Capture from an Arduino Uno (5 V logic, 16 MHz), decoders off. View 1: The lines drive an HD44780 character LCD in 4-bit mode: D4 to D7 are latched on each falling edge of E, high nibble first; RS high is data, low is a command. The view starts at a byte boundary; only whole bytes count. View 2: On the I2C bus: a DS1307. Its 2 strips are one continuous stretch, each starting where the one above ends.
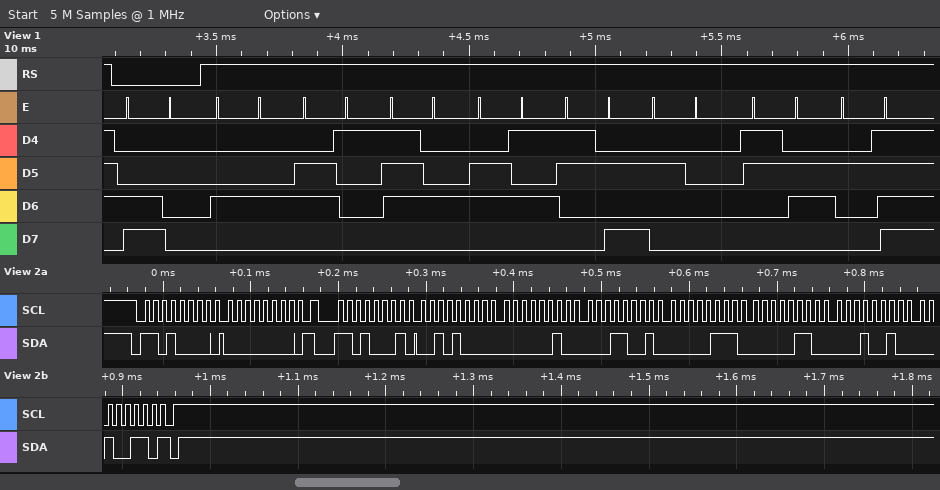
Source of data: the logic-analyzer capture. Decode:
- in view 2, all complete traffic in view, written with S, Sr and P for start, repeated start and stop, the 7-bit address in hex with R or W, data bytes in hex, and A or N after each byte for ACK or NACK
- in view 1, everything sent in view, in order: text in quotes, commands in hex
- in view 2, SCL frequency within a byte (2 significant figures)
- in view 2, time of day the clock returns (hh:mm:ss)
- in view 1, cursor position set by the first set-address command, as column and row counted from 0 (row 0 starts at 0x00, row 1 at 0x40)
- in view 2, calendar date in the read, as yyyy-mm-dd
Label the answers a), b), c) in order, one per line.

a) S 68W A 00 A Sr 68R A 28 A 02 A 19 A 07 A 06 A 12 A 26 N P
b) 0xC0 "Date: 6/"
c) 100 kHz
d) 19:02:28
e) column 0, row 1
f) 2026-12-06
